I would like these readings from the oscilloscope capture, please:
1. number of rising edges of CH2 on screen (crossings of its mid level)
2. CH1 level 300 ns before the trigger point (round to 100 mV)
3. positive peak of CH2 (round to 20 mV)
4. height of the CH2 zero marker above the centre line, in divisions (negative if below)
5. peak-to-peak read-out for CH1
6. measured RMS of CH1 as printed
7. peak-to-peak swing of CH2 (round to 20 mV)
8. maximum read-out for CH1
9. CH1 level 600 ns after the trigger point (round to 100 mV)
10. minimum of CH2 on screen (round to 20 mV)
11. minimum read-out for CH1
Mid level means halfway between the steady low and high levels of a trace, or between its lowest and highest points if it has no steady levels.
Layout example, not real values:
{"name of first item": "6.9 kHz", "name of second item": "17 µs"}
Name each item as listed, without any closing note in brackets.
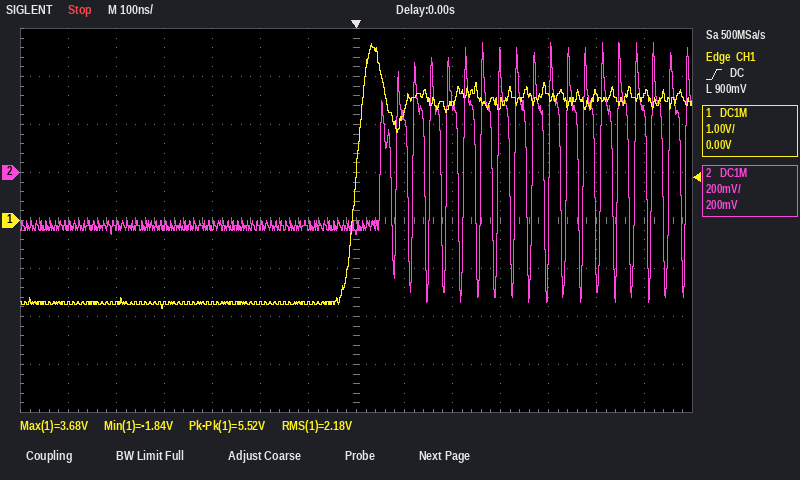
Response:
{"number of rising edges of CH2 on screen": "19", "CH1 level 300 ns before the trigger point": "-1.7 V", "positive peak of CH2": "540 mV", "height of the CH2 zero marker above the centre line, in divisions": "+1.0 div", "peak-to-peak read-out for CH1": "5.52 V", "measured RMS of CH1 as printed": "2.18 V", "peak-to-peak swing of CH2": "1.08 V", "maximum read-out for CH1": "3.68 V", "CH1 level 600 ns after the trigger point": "2.6 V", "minimum of CH2 on screen": "-540 mV", "minimum read-out for CH1": "-1.84 V"}
